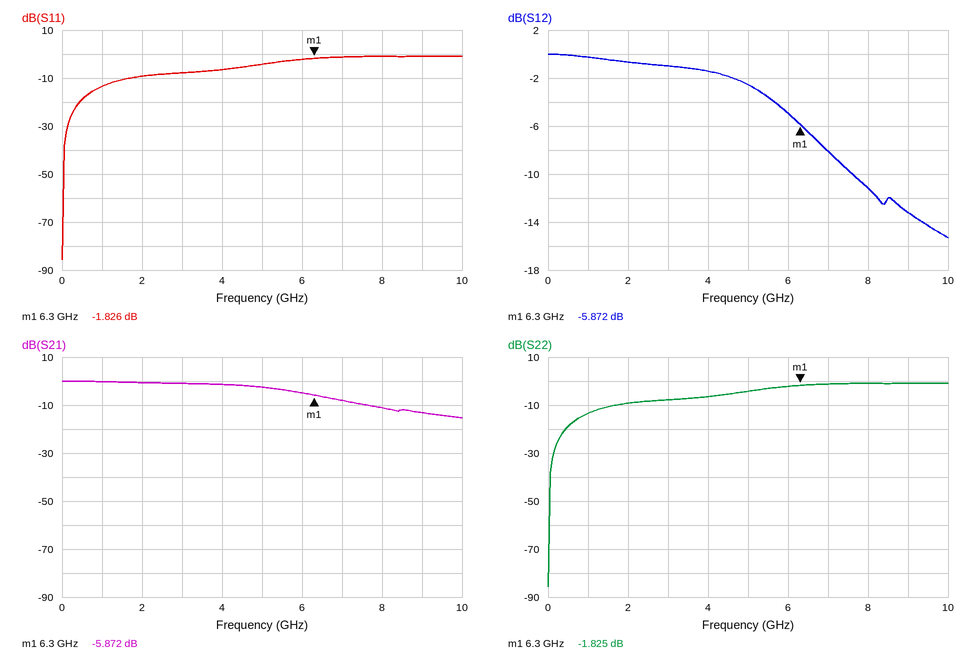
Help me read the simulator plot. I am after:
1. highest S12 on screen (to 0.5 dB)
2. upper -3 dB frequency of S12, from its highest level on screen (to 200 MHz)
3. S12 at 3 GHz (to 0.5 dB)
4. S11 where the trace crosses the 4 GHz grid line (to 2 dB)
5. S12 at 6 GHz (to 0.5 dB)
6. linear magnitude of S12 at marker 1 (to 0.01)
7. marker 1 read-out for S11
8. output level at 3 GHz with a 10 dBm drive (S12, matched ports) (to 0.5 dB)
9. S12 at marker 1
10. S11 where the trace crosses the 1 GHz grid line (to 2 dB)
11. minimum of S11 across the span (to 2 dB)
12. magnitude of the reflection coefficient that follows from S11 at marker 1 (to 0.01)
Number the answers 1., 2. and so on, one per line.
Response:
1. 0.0 dB
2. 5.2 GHz
3. -1.0 dB
4. -6 dB
5. -5.0 dB
6. 0.51
7. -1.826 dB
8. 9.0 dBm
9. -5.872 dB
10. -14 dB
11. -86 dB
12. 0.81
